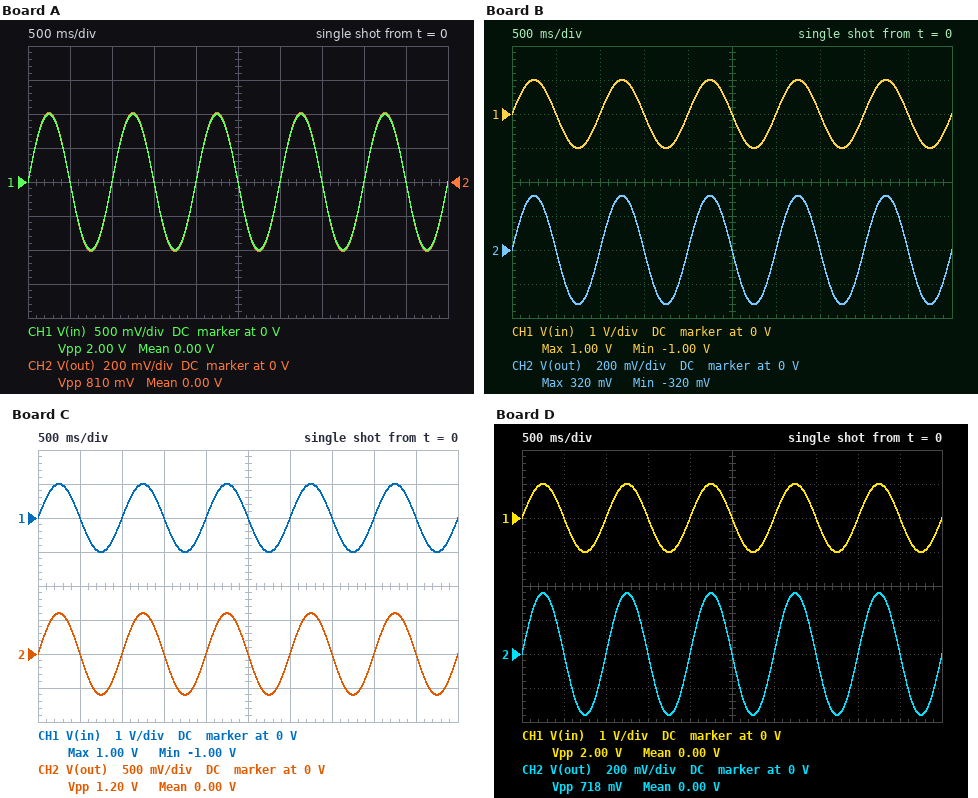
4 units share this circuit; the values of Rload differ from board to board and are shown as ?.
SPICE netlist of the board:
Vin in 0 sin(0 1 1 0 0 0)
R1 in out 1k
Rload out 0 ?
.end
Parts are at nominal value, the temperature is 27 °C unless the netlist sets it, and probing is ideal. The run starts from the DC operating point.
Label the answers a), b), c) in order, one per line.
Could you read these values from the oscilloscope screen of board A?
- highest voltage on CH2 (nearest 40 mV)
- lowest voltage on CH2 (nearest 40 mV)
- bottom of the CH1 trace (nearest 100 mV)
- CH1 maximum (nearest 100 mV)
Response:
a) 400 mV
b) -400 mV
c) -1.0 V
d) 1.0 V
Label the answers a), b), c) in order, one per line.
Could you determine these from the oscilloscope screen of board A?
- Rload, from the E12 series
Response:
a) 680 Ω
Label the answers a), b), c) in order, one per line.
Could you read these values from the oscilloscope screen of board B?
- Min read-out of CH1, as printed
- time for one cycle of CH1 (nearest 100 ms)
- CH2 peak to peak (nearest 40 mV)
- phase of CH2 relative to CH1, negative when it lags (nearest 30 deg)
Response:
a) -1.00 V
b) 1.0 s
c) 640 mV
d) 0 deg
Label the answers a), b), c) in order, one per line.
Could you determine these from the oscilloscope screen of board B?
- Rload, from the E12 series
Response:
a) 470 Ω
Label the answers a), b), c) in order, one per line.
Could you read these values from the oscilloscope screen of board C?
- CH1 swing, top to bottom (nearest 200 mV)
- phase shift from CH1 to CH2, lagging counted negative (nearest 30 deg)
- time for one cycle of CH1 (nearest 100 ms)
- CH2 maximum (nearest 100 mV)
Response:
a) 2.0 V
b) 0 deg
c) 1.0 s
d) 600 mV
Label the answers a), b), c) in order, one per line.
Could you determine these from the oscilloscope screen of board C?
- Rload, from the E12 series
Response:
a) 1.5 kΩ
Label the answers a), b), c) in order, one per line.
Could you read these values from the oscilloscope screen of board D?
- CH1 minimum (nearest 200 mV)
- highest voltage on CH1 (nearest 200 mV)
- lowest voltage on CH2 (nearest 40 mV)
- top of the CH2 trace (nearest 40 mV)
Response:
a) -1.0 V
b) 1.0 V
c) -360 mV
d) 360 mV
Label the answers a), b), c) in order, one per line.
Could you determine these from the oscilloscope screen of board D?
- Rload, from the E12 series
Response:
a) 560 Ω
